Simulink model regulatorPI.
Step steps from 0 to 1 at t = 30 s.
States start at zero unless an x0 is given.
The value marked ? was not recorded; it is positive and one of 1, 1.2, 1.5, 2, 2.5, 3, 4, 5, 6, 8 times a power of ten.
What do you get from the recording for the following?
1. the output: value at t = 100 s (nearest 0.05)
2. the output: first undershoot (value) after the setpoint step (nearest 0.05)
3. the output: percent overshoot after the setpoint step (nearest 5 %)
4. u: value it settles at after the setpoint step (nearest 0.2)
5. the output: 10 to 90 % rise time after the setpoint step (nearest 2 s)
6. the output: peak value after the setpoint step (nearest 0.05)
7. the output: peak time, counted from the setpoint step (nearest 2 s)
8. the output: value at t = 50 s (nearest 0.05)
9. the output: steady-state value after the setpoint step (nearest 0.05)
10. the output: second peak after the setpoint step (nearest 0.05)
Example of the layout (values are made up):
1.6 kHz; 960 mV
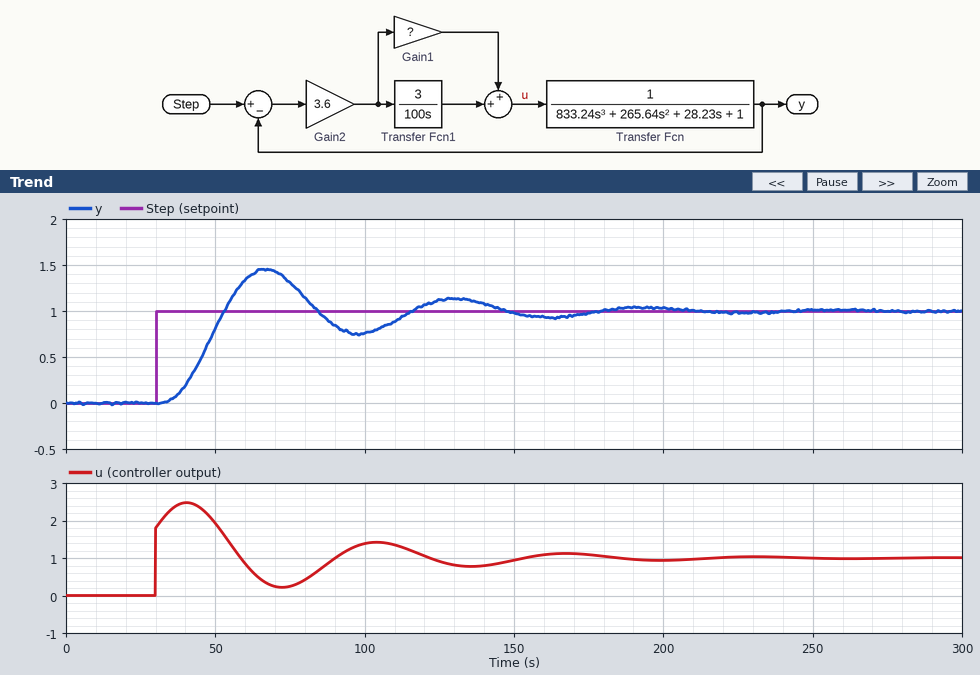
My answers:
0.75; 0.75; 45 %; 1.0; 14 s; 1.45; 36 s; 0.80; 1.00; 1.15
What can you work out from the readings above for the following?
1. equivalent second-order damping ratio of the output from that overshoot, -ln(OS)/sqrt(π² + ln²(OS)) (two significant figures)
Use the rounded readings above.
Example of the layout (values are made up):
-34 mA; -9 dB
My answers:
0.25
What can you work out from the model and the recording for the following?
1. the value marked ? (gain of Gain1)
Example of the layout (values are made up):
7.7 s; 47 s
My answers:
0.5
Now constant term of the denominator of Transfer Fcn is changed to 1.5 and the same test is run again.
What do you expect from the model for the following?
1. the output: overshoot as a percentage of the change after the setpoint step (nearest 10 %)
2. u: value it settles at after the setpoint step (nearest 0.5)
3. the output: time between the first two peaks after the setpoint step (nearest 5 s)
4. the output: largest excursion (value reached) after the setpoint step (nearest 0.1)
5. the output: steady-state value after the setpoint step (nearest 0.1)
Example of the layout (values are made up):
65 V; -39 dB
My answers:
30 %; 1.5; 55 s; 1.3; 1.0
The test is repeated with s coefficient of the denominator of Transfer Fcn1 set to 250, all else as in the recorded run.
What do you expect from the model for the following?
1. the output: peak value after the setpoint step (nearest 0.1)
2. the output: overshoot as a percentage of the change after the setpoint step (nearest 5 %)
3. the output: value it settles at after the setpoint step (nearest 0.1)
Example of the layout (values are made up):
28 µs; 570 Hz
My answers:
1.1; 10 %; 1.0
